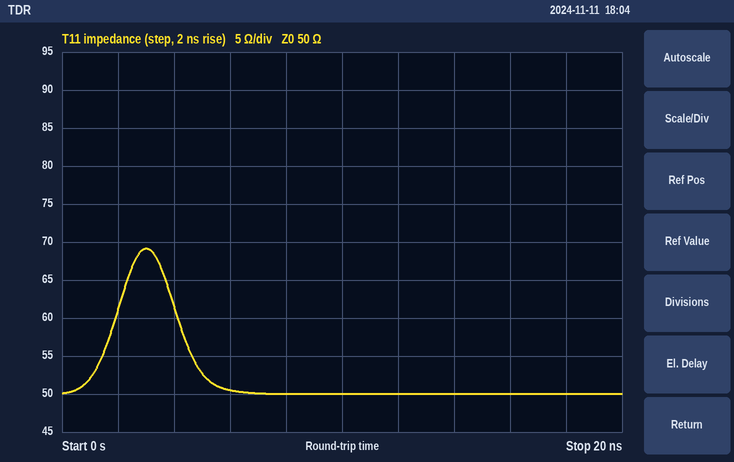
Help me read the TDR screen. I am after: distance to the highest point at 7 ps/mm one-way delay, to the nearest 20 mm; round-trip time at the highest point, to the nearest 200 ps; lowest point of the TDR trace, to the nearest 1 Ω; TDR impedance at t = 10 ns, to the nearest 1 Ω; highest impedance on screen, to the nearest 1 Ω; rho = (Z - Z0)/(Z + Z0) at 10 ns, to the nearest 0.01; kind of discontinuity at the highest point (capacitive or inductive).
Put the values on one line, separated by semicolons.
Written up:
220 mm; 3.0 ns; 50 Ω; 50 Ω; 69 Ω; 0.00; inductive
